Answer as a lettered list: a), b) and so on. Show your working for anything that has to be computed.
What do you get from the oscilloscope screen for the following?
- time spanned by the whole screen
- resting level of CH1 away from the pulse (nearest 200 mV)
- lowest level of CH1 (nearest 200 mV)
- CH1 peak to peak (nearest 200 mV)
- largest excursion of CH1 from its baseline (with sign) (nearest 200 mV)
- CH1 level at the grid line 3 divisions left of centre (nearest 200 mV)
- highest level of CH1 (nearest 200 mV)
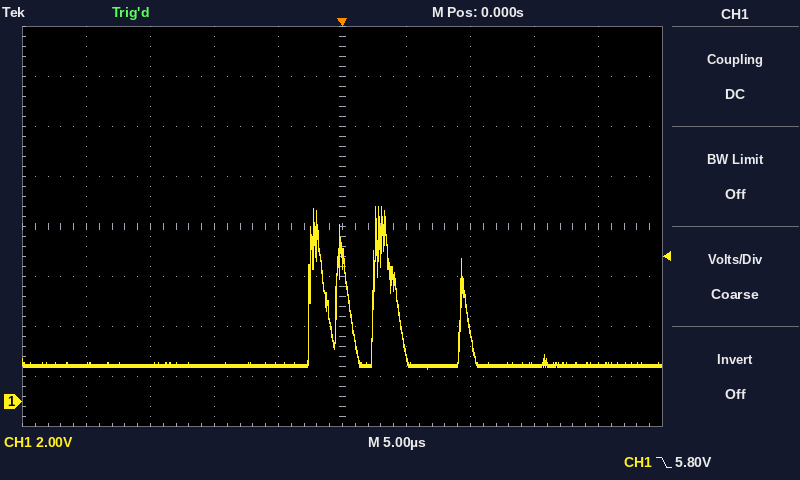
a) 50 µs
b) 1.4 V
c) 1.4 V
d) 7.8 V − (1.4 V) = 6.4 V
e) 7.8 V − (1.4 V) = +6.4 V
f) 1.4 V
g) 7.8 V
